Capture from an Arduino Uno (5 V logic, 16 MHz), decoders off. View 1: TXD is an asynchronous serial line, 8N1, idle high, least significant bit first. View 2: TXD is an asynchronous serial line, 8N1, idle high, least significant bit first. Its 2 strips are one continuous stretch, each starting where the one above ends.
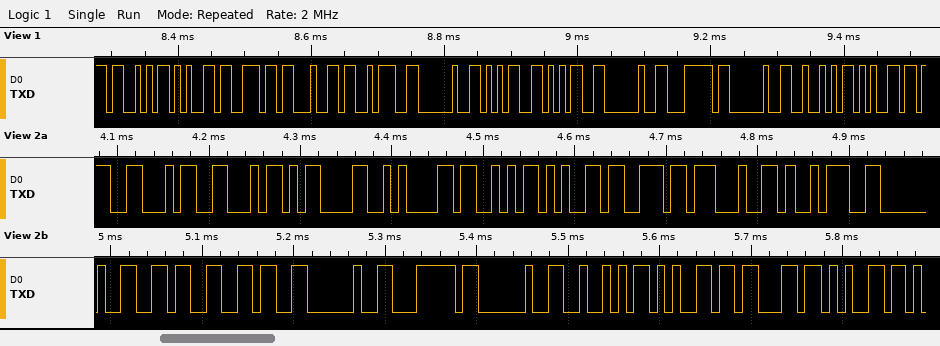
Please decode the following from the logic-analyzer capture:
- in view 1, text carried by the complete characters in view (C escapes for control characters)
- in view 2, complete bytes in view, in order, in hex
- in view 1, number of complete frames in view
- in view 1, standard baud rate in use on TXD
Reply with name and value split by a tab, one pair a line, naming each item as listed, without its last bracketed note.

in view 1, text carried by the complete characters in view	"Send: 55 | Re"
in view 2, complete bytes in view, in order, in hex	46 46 0D 0A 53 65 6E 64 3A 20 36 36 20 7C 20 52 65 63 65
in view 1, number of complete frames in view	13
in view 1, standard baud rate in use on TXD	115200 baud
